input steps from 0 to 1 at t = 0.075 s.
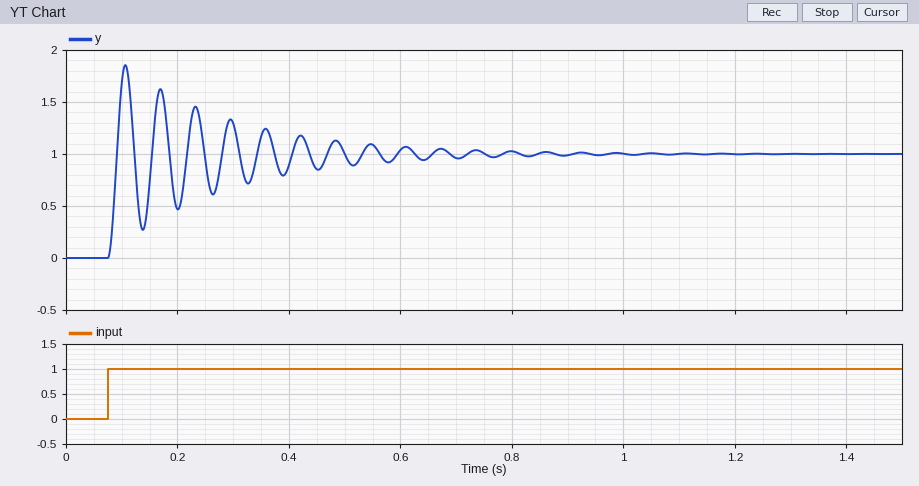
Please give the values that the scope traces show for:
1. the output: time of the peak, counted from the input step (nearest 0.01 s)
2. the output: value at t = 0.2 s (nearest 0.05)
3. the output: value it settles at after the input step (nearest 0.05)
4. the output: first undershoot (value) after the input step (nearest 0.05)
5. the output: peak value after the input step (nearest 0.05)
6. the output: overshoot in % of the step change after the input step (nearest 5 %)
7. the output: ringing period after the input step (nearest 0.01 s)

0.03 s
0.45
1.00
0.25
1.85
85 %
0.06 s
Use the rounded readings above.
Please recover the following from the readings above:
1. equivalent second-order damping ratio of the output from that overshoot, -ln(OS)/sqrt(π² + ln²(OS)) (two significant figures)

0.052
